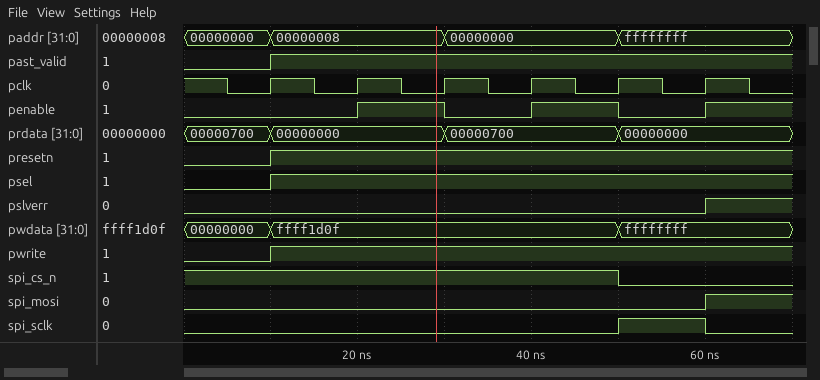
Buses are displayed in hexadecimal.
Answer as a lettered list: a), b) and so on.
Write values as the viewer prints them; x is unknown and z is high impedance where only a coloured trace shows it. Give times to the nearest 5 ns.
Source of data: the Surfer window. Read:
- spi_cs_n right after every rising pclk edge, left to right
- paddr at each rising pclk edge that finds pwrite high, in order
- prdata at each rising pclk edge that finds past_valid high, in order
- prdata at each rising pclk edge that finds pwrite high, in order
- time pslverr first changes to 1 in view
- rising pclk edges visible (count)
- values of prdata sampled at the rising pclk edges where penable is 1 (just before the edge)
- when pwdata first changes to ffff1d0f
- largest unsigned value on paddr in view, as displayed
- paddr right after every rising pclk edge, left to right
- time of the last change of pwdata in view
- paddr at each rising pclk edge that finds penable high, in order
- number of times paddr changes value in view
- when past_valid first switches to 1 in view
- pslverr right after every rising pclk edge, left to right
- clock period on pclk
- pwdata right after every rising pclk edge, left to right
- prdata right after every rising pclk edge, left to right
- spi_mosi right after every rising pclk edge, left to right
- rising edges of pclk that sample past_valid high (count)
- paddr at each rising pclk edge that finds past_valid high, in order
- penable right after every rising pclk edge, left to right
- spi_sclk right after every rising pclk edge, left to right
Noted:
a) 1 1 1 1 0 0
b) 00000008, 00000008, 00000000, 00000000, ffffffff
c) 00000000, 00000000, 00000700, 00000700, 00000000
d) 00000000, 00000000, 00000700, 00000700, 00000000
e) 60 ns
f) 6
g) 00000000, 00000700
h) 10 ns
i) ffffffff
j) 00000008, 00000008, 00000000, 00000000, ffffffff, ffffffff
k) 50 ns
l) 00000008, 00000000
m) 3
n) 10 ns
o) 0 0 0 0 0 1
p) 10 ns
q) ffff1d0f, ffff1d0f, ffff1d0f, ffff1d0f, ffffffff, ffffffff
r) 00000000, 00000000, 00000700, 00000700, 00000000, 00000000
s) 0 0 0 0 0 1
t) 5
u) 00000008, 00000008, 00000000, 00000000, ffffffff
v) 0 1 0 1 0 1
w) 0 0 0 0 1 0
